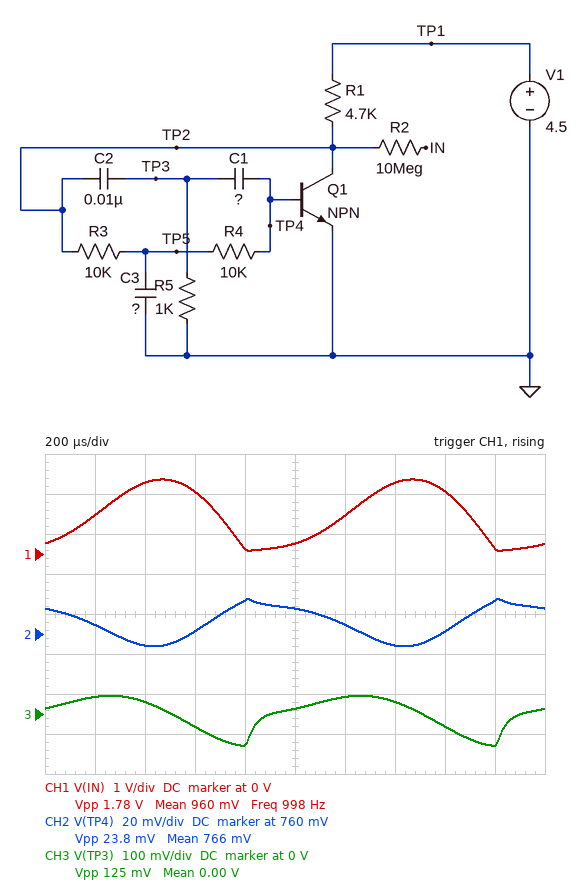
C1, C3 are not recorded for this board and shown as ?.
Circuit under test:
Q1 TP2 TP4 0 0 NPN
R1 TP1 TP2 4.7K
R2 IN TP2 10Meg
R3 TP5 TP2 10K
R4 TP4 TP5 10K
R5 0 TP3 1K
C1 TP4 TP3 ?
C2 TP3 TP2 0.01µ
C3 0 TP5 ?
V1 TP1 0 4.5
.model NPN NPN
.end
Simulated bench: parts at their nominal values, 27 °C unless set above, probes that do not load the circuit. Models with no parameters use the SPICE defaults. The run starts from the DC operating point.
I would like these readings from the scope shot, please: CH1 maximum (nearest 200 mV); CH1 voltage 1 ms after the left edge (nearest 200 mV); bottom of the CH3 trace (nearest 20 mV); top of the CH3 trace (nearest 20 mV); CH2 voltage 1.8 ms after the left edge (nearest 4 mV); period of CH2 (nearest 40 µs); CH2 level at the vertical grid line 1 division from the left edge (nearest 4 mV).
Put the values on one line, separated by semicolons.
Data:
1.8 V; 200 mV; -80 mV; 40 mV; 776 mV; 1.00 ms; 764 mV
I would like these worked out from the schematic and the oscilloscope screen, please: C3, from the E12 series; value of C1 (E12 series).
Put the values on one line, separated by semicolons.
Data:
180 nF; 27 nF
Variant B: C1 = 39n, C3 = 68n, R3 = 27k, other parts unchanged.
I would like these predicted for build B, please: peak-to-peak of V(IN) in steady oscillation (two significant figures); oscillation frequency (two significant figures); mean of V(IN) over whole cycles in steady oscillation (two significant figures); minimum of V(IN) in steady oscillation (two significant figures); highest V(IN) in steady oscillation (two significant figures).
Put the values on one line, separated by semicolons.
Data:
2.1 V; 870 Hz; 1.1 V; 79 mV; 2.2 V
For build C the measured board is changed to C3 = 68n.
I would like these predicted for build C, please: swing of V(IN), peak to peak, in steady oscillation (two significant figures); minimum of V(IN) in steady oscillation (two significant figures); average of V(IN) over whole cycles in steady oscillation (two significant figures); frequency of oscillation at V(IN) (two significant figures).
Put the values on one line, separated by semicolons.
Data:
2.0 V; 70 mV; 1.0 V; 1.3 kHz
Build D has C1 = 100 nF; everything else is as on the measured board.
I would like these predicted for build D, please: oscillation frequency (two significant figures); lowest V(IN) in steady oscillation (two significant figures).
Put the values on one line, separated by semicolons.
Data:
630 Hz; 91 mV
